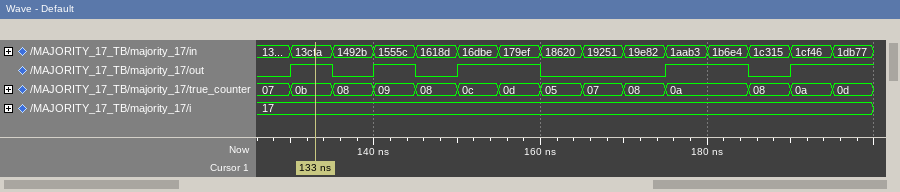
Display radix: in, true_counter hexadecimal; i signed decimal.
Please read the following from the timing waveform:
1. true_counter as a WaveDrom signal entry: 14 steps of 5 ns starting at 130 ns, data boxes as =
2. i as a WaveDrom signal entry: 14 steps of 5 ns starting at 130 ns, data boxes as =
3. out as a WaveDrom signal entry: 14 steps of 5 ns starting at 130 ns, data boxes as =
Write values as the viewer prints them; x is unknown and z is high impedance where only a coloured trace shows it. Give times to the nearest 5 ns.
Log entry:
{name: 'true_counter', wave: '==========.===', data: '0b 08 09 08 0c 0d 05 07 08 0a 08 0a 0d'}
{name: 'i', wave: '=.............', data: '17'}
{name: 'out', wave: '10101.0..1.01.'}
